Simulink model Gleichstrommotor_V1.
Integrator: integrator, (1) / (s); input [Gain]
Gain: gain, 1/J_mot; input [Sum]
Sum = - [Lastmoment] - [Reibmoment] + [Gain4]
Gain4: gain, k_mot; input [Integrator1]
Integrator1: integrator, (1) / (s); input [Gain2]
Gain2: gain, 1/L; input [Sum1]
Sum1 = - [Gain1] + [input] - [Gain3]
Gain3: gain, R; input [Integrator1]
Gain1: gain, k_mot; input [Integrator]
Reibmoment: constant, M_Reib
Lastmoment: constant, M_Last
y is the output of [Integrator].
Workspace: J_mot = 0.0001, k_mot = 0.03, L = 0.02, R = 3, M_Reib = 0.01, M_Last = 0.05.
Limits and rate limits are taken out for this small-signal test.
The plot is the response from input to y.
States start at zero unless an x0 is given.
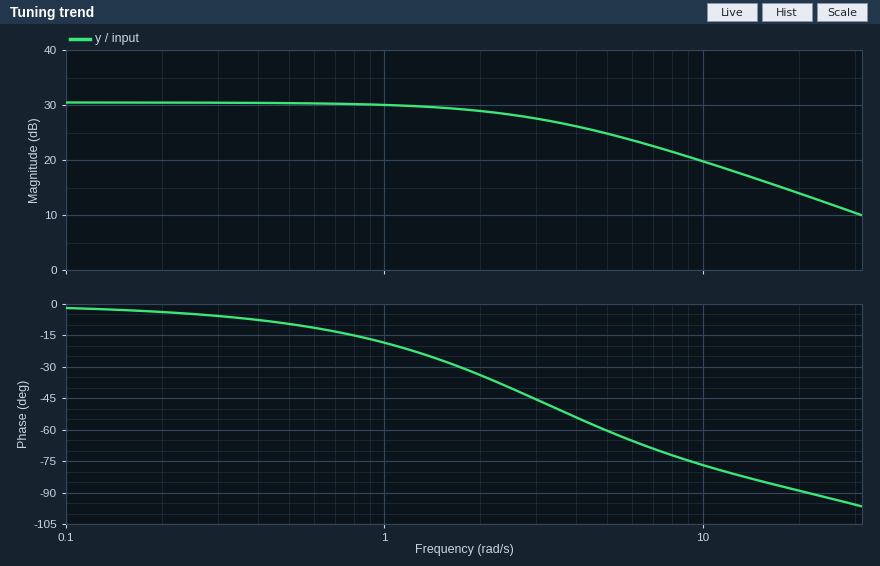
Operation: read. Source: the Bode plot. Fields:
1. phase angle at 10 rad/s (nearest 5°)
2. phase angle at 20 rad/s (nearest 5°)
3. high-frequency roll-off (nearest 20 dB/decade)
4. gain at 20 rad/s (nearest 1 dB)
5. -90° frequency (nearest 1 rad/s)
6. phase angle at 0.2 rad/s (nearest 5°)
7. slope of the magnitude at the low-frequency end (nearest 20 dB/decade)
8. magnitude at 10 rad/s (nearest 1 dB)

-75°
-90°
-20 dB/decade
14 dB
21 rad/s
-5°
0 dB/decade
20 dB
